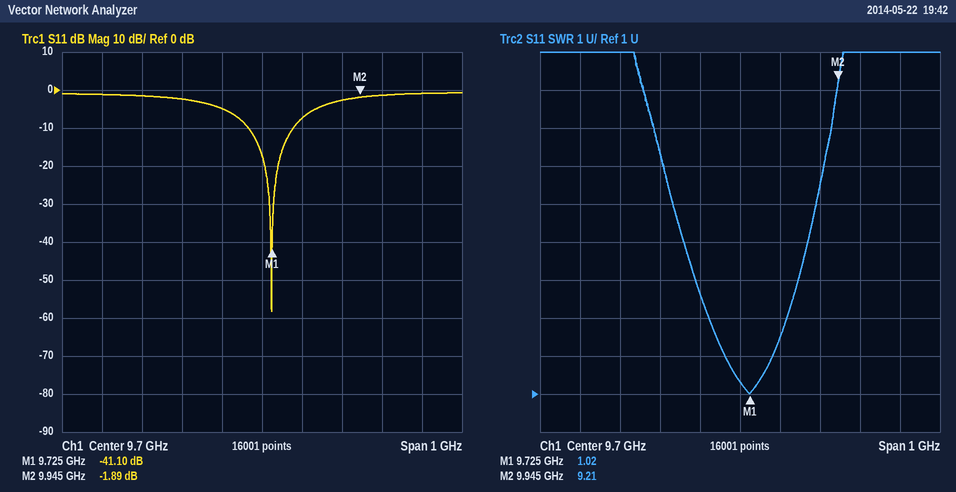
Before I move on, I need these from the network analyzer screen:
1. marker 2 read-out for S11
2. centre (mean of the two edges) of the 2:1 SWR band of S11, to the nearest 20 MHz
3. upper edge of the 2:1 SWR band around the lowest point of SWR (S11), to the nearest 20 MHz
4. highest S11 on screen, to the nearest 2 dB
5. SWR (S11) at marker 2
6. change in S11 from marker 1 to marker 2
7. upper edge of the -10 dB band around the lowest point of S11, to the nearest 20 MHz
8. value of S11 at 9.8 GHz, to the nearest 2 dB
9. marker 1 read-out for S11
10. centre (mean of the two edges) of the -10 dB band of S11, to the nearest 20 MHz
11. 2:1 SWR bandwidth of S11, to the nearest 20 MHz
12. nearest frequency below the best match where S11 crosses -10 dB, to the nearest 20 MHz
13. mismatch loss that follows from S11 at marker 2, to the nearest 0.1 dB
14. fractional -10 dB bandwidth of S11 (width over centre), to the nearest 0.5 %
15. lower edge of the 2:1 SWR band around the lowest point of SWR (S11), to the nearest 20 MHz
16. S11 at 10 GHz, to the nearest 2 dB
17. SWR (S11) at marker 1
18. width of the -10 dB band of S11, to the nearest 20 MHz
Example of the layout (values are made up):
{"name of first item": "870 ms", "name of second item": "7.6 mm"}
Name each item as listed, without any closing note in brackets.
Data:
{"marker 2 read-out for S11": "-1.89 dB", "centre (mean of the two edges) of the 2:1 SWR band of S11, to the nearest 20 MHz": "9.72 GHz", "upper edge of the 2:1 SWR band around the lowest point of SWR (S11), to the nearest 20 MHz": "9.78 GHz", "highest S11 on screen, to the nearest 2 dB": "0 dB", "SWR (S11) at marker 2": "9.21", "change in S11 from marker 1 to marker 2": "39.21 dB", "upper edge of the -10 dB band around the lowest point of S11, to the nearest 20 MHz": "9.78 GHz", "value of S11 at 9.8 GHz, to the nearest 2 dB": "-8 dB", "marker 1 read-out for S11": "-41.10 dB", "centre (mean of the two edges) of the -10 dB band of S11, to the nearest 20 MHz": "9.72 GHz", "2:1 SWR bandwidth of S11, to the nearest 20 MHz": "120 MHz", "nearest frequency below the best match where S11 crosses -10 dB, to the nearest 20 MHz": "9.66 GHz", "mismatch loss that follows from S11 at marker 2, to the nearest 0.1 dB": "4.5 dB", "fractional -10 dB bandwidth of S11 (width over centre), to the nearest 0.5 %": "1.0 %", "lower edge of the 2:1 SWR band around the lowest point of SWR (S11), to the nearest 20 MHz": "9.66 GHz", "S11 at 10 GHz, to the nearest 2 dB": "-2 dB", "SWR (S11) at marker 1": "1.02", "width of the -10 dB band of S11, to the nearest 20 MHz": "120 MHz"}
